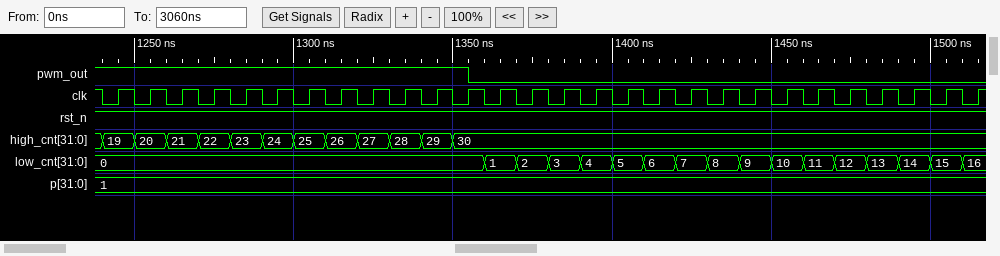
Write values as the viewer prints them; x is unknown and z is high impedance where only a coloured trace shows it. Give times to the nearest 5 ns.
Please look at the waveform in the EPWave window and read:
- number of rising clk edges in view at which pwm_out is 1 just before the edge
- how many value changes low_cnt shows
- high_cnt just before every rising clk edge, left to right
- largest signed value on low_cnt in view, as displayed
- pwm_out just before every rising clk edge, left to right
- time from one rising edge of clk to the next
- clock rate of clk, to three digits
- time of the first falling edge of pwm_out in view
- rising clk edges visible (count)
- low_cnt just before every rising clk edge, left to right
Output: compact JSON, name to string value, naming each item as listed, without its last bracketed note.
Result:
{"number of rising clk edges in view at which pwm_out is 1 just before the edge": "12", "how many value changes low_cnt shows": "16", "high_cnt just before every rising clk edge, left to right": "19, 20, 21, 22, 23, 24, 25, 26, 27, 28, 29, 30, 30, 30, 30, 30, 30, 30, 30, 30, 30, 30, 30, 30, 30, 30, 30, 30", "largest signed value on low_cnt in view, as displayed": "16", "pwm_out just before every rising clk edge, left to right": "1 1 1 1 1 1 1 1 1 1 1 1 0 0 0 0 0 0 0 0 0 0 0 0 0 0 0 0", "time from one rising edge of clk to the next": "10 ns", "clock rate of clk, to three digits": "100 MHz", "time of the first falling edge of pwm_out in view": "1355 ns", "rising clk edges visible": "28", "low_cnt just before every rising clk edge, left to right": "0, 0, 0, 0, 0, 0, 0, 0, 0, 0, 0, 0, 1, 2, 3, 4, 5, 6, 7, 8, 9, 10, 11, 12, 13, 14, 15, 16"}
